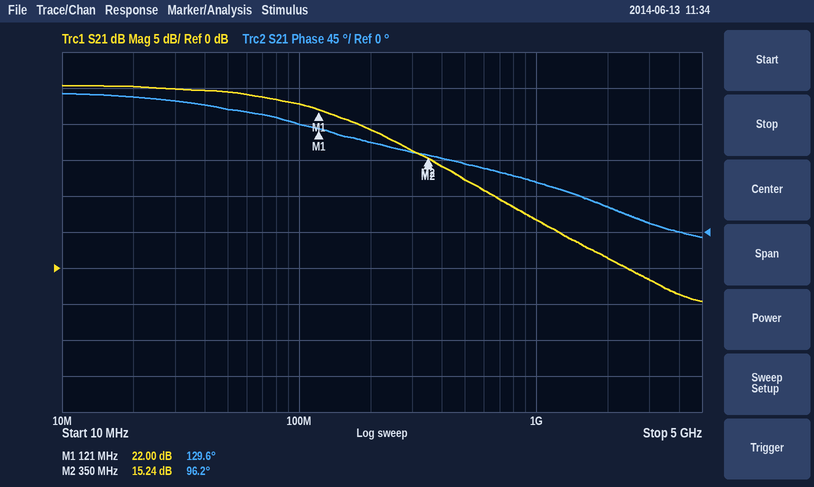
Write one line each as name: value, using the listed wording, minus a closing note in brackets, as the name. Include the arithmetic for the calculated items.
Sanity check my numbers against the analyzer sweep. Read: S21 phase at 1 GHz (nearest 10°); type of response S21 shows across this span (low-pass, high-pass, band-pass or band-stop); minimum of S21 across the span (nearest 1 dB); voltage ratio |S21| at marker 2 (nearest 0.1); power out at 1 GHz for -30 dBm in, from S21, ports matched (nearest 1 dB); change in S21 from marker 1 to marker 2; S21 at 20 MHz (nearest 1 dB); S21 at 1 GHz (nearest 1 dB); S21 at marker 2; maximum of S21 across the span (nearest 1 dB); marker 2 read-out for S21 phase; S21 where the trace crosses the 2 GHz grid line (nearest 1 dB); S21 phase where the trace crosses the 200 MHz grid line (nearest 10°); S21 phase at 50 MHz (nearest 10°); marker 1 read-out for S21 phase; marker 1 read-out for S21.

S21 phase at 1 GHz: 60°
type of response S21 shows across this span: low-pass
minimum of S21 across the span: -5 dB
voltage ratio |S21| at marker 2: 10^(15.24/20) ≈ 5.8
power out at 1 GHz for -30 dBm in, from S21, ports matched: -30 dBm + (7 dB) = -23 dBm
change in S21 from marker 1 to marker 2: 15.24 − (22) = -6.76 dB
S21 at 20 MHz: 25 dB
S21 at 1 GHz: 7 dB
S21 at marker 2: 15.24 dB
maximum of S21 across the span: 25 dB
marker 2 read-out for S21 phase: 96.2°
S21 where the trace crosses the 2 GHz grid line: 1 dB
S21 phase where the trace crosses the 200 MHz grid line: 110°
S21 phase at 50 MHz: 150°
marker 1 read-out for S21 phase: 129.6°
marker 1 read-out for S21: 22.00 dB
